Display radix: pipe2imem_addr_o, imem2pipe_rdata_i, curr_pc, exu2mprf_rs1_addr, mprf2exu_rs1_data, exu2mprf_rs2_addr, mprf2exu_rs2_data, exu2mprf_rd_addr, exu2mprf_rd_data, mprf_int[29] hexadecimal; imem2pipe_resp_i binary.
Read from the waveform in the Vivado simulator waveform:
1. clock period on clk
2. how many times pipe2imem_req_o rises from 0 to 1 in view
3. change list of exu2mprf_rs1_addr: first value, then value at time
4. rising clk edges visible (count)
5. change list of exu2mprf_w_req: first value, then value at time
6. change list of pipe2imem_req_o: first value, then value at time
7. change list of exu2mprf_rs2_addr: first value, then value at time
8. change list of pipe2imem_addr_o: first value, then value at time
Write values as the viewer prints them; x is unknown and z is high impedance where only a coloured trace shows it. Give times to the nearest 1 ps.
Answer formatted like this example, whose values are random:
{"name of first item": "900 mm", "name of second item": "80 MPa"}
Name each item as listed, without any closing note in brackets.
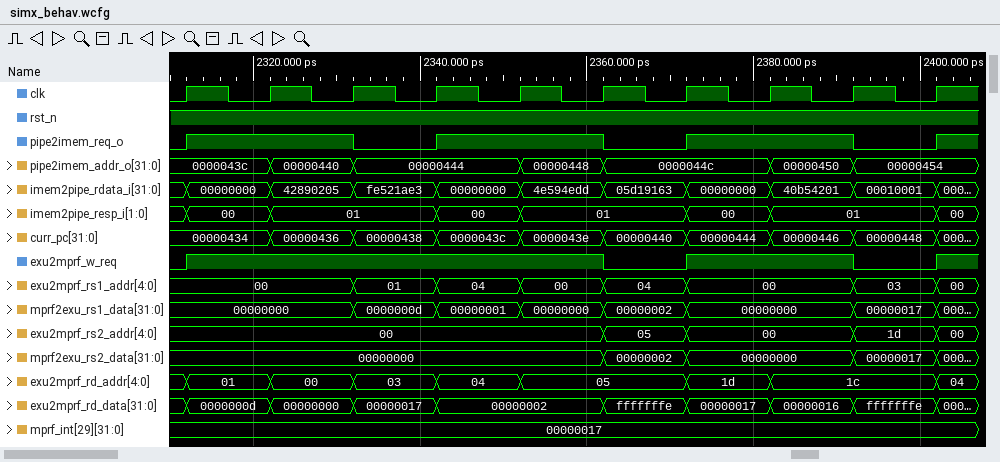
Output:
{"clock period on clk": "10 ps", "how many times pipe2imem_req_o rises from 0 to 1 in view": "4", "change list of exu2mprf_rs1_addr: first value, then value at time": "00, 01 at 2332 ps, 04 at 2342 ps, 00 at 2352 ps, 04 at 2362 ps, 00 at 2372 ps, 03 at 2392 ps, 00 at 2402 ps", "rising clk edges visible": "10", "change list of exu2mprf_w_req: first value, then value at time": "0, 1 at 2312 ps, 0 at 2362 ps, 1 at 2372 ps, 0 at 2392 ps, 1 at 2402 ps", "change list of pipe2imem_req_o: first value, then value at time": "0, 1 at 2312 ps, 0 at 2332 ps, 1 at 2342 ps, 0 at 2362 ps, 1 at 2372 ps, 0 at 2392 ps, 1 at 2402 ps", "change list of exu2mprf_rs2_addr: first value, then value at time": "00, 05 at 2362 ps, 00 at 2372 ps, 1d at 2392 ps, 00 at 2402 ps", "change list of pipe2imem_addr_o: first value, then value at time": "0000043c, 00000440 at 2322 ps, 00000444 at 2332 ps, 00000448 at 2352 ps, 0000044c at 2362 ps, 00000450 at 2382 ps, 00000454 at 2392 ps"}
